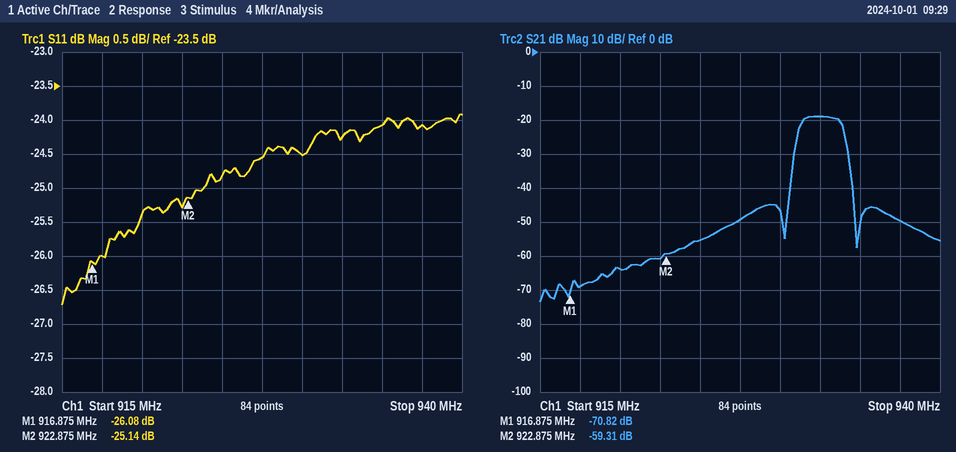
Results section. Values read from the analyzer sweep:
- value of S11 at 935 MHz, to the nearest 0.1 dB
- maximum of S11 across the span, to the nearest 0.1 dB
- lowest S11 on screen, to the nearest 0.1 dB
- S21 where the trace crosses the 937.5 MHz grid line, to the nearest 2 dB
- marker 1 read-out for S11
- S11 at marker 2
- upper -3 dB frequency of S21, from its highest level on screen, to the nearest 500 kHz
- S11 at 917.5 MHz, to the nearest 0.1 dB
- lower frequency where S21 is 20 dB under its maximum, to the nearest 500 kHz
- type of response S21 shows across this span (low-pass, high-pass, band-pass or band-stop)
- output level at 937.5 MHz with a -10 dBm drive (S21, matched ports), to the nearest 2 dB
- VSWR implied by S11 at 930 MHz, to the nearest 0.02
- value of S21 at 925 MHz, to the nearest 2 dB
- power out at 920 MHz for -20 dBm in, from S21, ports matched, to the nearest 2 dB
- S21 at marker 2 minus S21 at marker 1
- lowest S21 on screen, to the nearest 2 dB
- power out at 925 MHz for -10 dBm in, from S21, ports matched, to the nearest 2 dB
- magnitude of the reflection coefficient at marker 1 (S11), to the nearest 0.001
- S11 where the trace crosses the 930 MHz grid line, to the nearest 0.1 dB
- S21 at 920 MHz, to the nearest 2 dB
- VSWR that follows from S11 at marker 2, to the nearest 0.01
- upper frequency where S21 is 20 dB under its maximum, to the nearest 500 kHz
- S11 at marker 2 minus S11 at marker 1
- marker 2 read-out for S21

-24.1 dB
-23.9 dB
-26.7 dB
-50 dB
-26.08 dB
-25.14 dB
934.0 MHz
-26.0 dB
930.5 MHz
band-pass
-60 dBm
1.12
-56 dB
-84 dBm
11.51 dB
-74 dB
-66 dBm
0.050
-24.5 dB
-64 dB
1.12
934.5 MHz
0.94 dB
-59.31 dB
